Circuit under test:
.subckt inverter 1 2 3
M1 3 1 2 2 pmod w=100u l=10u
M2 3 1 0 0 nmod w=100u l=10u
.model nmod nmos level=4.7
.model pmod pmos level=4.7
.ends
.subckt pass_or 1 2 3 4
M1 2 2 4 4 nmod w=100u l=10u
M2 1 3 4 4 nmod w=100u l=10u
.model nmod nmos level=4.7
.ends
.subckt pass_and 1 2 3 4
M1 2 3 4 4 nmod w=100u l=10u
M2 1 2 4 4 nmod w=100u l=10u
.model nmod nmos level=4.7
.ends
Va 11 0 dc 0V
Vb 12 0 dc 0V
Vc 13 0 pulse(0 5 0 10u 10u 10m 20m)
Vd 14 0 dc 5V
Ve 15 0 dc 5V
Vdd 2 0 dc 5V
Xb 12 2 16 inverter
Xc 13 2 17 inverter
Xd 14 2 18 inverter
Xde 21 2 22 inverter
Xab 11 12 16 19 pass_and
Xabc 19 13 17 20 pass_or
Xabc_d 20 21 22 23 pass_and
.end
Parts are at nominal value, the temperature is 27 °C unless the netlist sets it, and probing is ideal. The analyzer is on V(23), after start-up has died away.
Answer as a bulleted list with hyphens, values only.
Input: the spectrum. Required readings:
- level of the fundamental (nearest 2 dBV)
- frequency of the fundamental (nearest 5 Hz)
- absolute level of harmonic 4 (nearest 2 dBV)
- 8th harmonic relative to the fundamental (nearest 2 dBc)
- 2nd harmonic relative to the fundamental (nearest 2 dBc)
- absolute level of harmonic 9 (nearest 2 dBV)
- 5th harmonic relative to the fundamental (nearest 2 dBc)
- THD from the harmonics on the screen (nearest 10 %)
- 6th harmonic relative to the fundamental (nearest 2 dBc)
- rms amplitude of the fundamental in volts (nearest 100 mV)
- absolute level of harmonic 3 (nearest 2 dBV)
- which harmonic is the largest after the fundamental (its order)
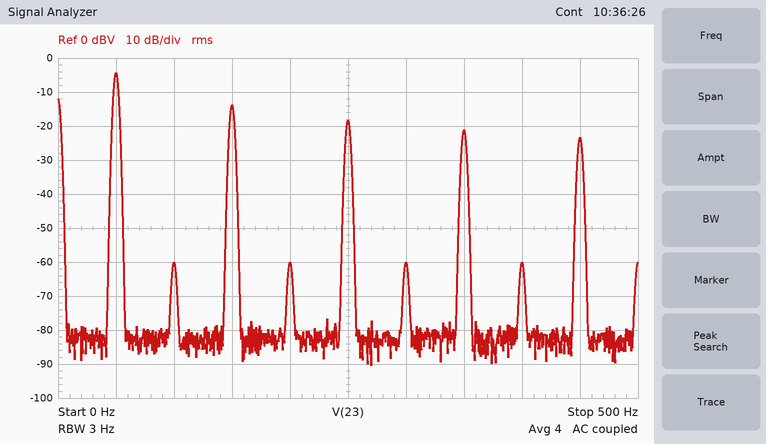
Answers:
- -4 dBV
- 50 Hz
- -60 dBV
- -56 dBc
- -56 dBc
- -24 dBV
- -14 dBc
- 40 %
- -56 dBc
- 600 mV
- -14 dBV
- 3
